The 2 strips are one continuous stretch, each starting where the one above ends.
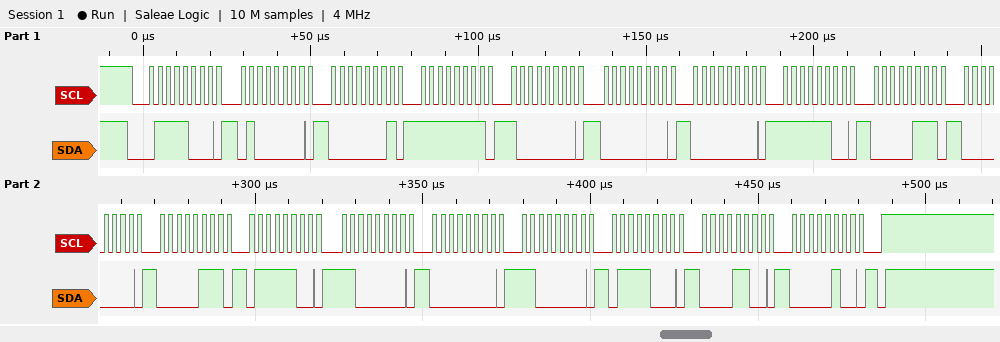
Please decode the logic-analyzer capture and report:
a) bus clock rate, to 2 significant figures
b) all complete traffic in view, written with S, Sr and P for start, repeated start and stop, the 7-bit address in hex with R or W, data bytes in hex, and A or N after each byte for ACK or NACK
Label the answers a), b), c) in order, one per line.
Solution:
a) 400 kHz
b) S 3CW A 40 A 01 A FF A 80 A 00 A 00 A FC A 07 A 00 A 07 A 7C A C0 A 00 A C0 A 78 A 0C A 04 A P
